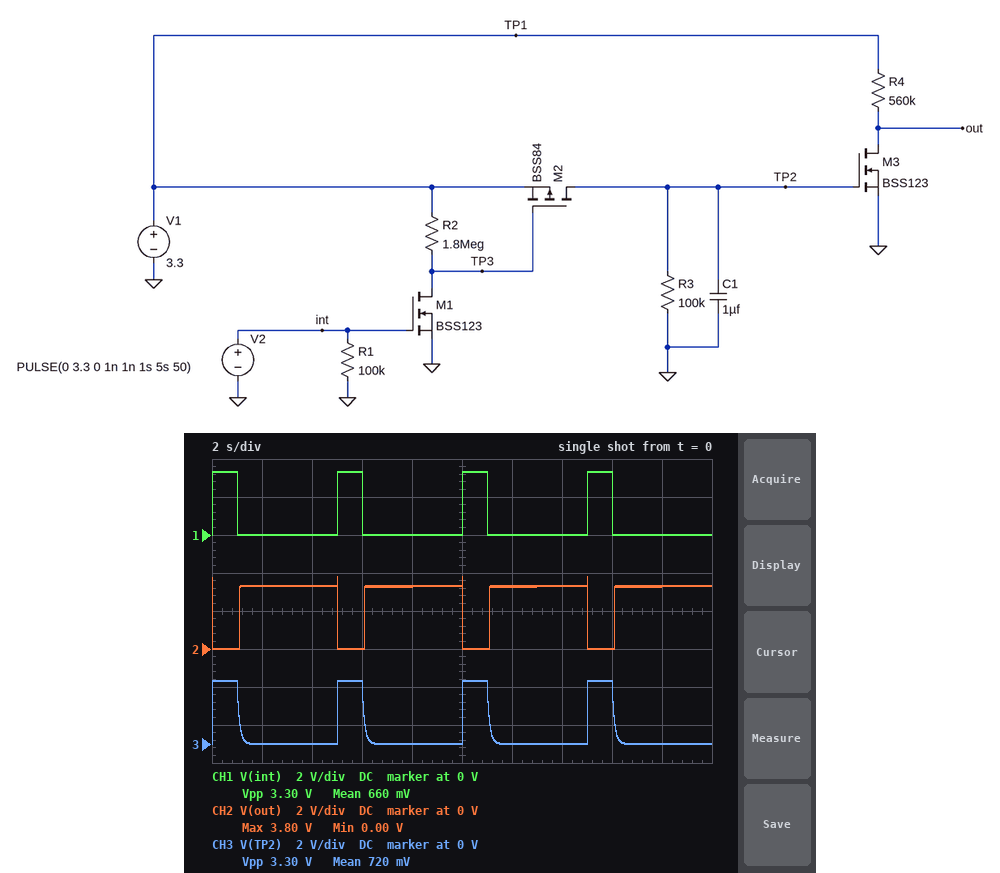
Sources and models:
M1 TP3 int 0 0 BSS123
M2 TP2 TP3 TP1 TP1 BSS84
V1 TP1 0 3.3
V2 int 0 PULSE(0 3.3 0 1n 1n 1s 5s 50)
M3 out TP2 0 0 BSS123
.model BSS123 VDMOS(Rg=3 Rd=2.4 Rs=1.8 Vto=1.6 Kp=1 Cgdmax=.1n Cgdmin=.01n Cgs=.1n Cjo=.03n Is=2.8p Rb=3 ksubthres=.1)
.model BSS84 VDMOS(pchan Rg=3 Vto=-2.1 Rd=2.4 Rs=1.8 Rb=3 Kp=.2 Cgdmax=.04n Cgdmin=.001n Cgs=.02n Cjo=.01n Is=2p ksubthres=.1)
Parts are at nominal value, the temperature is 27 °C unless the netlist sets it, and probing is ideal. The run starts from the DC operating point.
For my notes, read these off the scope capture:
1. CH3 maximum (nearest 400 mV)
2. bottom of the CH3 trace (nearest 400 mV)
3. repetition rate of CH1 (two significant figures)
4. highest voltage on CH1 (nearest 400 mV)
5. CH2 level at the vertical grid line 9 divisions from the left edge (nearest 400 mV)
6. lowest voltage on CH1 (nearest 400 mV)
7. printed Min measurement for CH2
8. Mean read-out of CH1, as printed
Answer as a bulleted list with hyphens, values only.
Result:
- 3.2 V
- 0 V
- 200 mHz
- 3.2 V
- 3.2 V
- 0 V
- 0.00 V
- 660 mV
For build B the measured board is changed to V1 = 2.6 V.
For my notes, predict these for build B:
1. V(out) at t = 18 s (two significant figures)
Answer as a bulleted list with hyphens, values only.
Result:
- 2.6 V
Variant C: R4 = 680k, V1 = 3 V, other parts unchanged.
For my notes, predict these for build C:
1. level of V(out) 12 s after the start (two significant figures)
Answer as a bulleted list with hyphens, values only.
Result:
- 3.0 V
